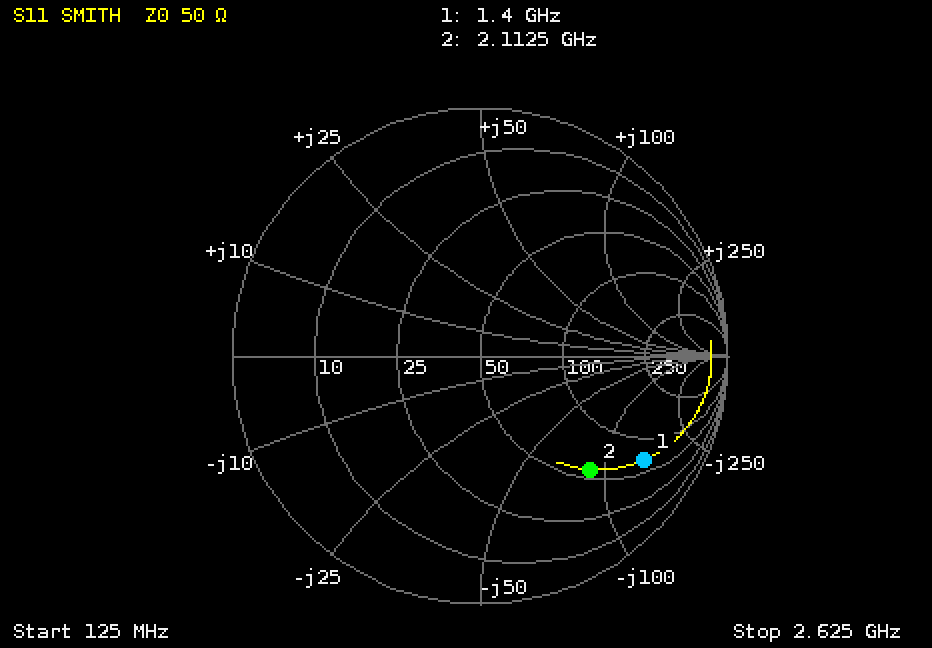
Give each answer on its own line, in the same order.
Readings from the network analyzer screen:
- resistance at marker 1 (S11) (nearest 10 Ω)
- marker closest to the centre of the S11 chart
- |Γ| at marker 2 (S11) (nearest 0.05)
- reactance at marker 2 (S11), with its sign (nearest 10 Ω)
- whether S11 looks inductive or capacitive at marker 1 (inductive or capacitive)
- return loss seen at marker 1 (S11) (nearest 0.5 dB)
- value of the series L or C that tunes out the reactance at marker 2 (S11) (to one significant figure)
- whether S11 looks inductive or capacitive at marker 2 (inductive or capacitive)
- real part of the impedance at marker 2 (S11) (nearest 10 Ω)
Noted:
70 Ω
marker 2
0.65
-90 Ω
capacitive
2.0 dB
7 nH
capacitive
60 Ω
